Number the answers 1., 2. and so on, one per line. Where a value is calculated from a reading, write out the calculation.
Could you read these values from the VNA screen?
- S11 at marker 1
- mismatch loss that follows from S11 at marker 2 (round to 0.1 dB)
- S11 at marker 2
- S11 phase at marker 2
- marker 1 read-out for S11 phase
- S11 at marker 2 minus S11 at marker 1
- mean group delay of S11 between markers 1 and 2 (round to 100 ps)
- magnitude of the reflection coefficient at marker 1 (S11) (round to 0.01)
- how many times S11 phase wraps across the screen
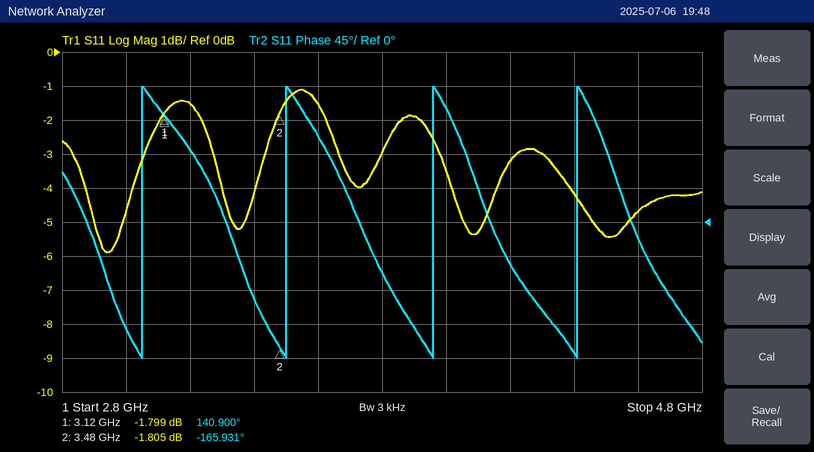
1. -1.799 dB
2. −10 log10(1 − 10^(-1.805/10)) ≈ 4.7 dB
3. -1.805 dB
4. -165.931°
5. 140.900°
6. -1.805 − (-1.799) = -0.006 dB
7. −(-165.931° − (140.9°))/(360° × 360 MHz) ≈ 2.4 ns
8. 10^(-1.799/20) ≈ 0.81
9. 4
